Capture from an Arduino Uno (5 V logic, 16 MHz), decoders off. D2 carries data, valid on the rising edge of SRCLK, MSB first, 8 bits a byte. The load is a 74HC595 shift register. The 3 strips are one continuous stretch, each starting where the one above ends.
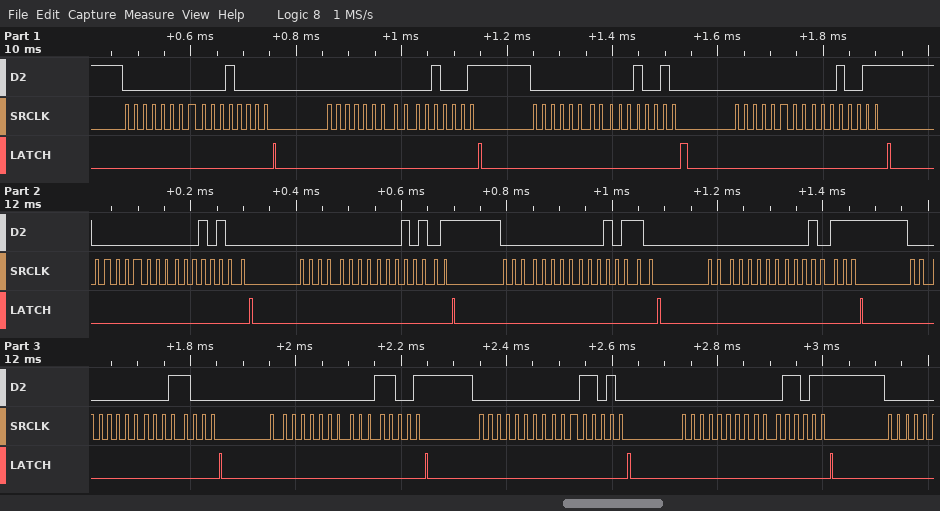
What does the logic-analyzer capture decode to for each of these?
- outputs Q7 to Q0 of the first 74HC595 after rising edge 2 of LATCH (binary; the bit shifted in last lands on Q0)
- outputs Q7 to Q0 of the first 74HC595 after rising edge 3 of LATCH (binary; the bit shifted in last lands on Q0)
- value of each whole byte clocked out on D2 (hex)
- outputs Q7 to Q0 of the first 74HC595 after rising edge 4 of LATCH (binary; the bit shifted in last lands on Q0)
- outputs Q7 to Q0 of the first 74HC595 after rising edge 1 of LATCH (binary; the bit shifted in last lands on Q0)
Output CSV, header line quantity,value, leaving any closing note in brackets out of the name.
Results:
quantity,value
outputs Q7 to Q0 of the first 74HC595 after rising edge 2 of LATCH,00010001
outputs Q7 to Q0 of the first 74HC595 after rising edge 3 of LATCH,00010010
value of each whole byte clocked out on D2,00 10 00 11 00 12 00 13 00 14 00 15 00 16 00 17 00 18 00 19 00 1A 00 1B
outputs Q7 to Q0 of the first 74HC595 after rising edge 4 of LATCH,00010011
outputs Q7 to Q0 of the first 74HC595 after rising edge 1 of LATCH,00010000
